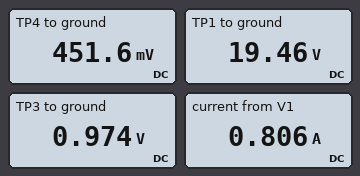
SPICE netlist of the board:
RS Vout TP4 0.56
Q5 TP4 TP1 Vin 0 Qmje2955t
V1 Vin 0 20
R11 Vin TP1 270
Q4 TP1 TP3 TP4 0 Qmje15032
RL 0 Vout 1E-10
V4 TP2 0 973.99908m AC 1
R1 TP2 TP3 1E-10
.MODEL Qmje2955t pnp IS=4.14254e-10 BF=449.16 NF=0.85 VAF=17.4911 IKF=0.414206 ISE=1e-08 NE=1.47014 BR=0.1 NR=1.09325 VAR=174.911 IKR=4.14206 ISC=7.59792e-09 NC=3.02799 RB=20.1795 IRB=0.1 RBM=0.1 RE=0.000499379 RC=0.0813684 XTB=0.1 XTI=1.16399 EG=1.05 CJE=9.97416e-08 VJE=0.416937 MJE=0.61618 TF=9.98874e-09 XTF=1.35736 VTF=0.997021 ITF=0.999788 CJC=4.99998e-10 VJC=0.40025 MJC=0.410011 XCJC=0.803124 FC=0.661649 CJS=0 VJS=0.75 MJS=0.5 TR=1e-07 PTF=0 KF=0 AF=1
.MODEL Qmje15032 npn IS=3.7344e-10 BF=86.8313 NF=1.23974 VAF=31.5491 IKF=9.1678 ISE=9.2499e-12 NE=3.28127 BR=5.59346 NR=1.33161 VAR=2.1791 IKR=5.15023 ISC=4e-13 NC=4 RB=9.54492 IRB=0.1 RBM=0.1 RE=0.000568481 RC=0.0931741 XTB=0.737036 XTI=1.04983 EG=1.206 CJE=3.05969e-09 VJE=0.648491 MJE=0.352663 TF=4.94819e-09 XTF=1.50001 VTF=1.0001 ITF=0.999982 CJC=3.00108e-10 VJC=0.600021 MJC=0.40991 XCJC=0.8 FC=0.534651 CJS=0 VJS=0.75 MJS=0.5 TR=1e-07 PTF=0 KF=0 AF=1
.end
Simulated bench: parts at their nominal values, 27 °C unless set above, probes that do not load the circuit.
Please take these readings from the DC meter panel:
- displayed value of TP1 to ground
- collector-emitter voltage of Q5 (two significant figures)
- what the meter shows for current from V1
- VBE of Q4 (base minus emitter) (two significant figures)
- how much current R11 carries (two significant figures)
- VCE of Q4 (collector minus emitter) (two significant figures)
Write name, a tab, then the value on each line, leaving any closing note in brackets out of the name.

displayed value of TP1 to ground	19.46 V
collector-emitter voltage of Q5	-20 V
what the meter shows for current from V1	0.806 A
VBE of Q4 (base minus emitter)	520 mV
how much current R11 carries	2.0 mA
VCE of Q4 (collector minus emitter)	19 V
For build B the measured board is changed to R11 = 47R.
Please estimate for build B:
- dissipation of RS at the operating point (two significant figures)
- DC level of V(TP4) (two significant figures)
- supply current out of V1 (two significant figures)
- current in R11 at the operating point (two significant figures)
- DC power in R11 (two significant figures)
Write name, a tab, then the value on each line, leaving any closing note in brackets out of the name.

dissipation of RS at the operating point	320 mW
DC level of V(TP4)	420 mV
supply current out of V1	750 mA
current in R11 at the operating point	11 mA
DC power in R11	6.0 mW
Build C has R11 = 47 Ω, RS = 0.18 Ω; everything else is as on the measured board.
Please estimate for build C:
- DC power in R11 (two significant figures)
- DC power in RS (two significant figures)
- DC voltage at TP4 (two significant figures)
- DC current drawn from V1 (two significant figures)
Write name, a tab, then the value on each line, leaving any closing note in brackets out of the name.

DC power in R11	11 mW
DC power in RS	880 mW
DC voltage at TP4	400 mV
DC current drawn from V1	2.2 A
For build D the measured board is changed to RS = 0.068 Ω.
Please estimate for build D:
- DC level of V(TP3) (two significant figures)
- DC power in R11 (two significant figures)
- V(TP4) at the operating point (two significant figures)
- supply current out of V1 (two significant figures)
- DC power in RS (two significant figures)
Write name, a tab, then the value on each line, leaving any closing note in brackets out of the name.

DC level of V(TP3)	970 mV
DC power in R11	5.6 mW
V(TP4) at the operating point	370 mV
supply current out of V1	5.4 A
DC power in RS	2.0 W
